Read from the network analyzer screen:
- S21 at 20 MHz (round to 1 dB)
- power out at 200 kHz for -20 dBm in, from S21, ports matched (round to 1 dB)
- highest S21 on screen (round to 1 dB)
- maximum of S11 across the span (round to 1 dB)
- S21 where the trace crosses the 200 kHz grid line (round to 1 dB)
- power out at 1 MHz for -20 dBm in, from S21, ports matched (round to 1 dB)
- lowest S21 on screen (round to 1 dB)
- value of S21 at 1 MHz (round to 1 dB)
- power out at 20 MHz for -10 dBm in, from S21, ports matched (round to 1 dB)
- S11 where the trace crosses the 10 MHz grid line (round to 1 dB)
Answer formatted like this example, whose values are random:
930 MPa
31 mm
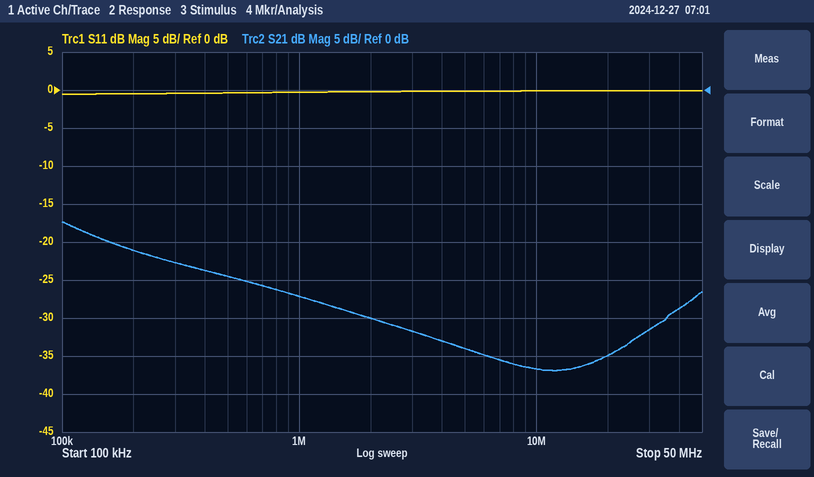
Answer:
-35 dB
-41 dBm
-17 dB
0 dB
-21 dB
-47 dBm
-37 dB
-27 dB
-45 dBm
0 dB
